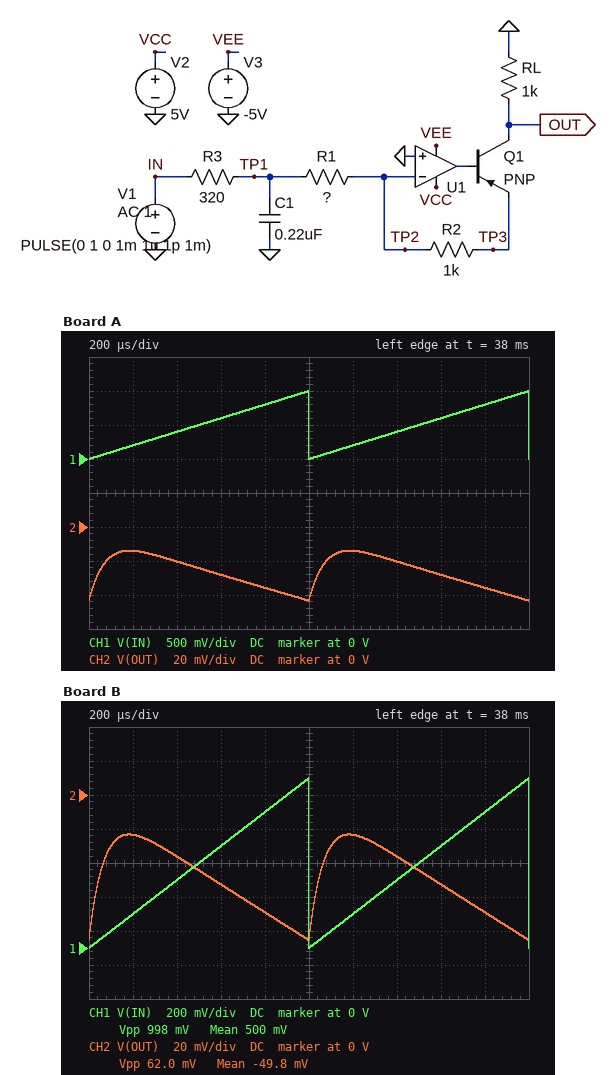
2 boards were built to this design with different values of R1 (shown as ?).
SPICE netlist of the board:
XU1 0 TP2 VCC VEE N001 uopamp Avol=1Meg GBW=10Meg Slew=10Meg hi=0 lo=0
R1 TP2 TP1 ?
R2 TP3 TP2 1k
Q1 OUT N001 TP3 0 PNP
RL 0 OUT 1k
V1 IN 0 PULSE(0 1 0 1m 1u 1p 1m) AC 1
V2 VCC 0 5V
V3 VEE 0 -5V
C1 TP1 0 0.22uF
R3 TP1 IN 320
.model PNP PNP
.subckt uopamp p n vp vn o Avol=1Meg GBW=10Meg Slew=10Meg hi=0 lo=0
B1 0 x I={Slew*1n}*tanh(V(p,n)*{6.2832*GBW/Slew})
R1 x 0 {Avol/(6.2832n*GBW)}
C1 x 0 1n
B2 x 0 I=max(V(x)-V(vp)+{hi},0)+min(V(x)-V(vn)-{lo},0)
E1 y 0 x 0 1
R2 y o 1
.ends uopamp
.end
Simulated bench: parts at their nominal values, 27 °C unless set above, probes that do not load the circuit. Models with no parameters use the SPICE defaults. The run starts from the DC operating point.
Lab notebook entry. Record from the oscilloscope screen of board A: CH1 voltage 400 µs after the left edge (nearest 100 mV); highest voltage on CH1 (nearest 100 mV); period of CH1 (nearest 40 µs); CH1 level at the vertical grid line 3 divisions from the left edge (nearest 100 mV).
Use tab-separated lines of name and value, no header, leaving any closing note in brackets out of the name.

CH1 voltage 400 µs after the left edge	400 mV
highest voltage on CH1	1.0 V
period of CH1	1.00 ms
CH1 level at the vertical grid line 3 divisions from the left edge	600 mV
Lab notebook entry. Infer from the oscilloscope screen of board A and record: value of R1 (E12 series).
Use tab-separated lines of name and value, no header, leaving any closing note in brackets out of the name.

value of R1	27 kΩ
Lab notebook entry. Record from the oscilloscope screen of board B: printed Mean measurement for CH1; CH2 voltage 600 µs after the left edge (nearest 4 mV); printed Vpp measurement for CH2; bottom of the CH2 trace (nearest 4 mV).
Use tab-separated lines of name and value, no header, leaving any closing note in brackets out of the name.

printed Mean measurement for CH1	500 mV
CH2 voltage 600 µs after the left edge	-52 mV
printed Vpp measurement for CH2	62.0 mV
bottom of the CH2 trace	-84 mV
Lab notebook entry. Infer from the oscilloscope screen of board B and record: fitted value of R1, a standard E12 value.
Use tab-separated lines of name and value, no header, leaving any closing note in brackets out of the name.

fitted value of R1, a standard E12 value	12 kΩ
